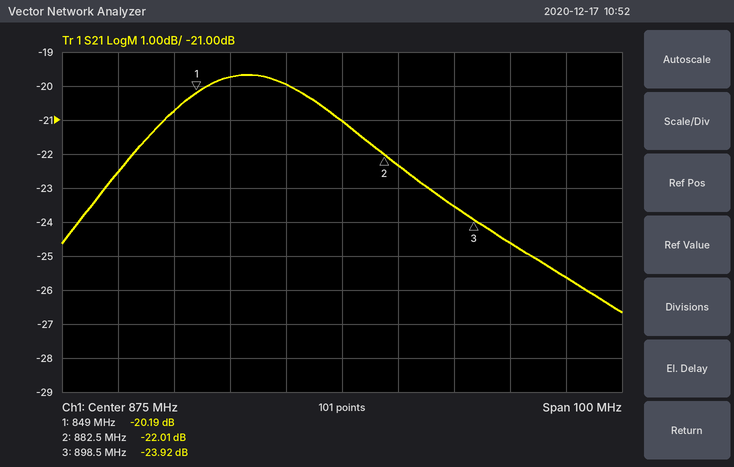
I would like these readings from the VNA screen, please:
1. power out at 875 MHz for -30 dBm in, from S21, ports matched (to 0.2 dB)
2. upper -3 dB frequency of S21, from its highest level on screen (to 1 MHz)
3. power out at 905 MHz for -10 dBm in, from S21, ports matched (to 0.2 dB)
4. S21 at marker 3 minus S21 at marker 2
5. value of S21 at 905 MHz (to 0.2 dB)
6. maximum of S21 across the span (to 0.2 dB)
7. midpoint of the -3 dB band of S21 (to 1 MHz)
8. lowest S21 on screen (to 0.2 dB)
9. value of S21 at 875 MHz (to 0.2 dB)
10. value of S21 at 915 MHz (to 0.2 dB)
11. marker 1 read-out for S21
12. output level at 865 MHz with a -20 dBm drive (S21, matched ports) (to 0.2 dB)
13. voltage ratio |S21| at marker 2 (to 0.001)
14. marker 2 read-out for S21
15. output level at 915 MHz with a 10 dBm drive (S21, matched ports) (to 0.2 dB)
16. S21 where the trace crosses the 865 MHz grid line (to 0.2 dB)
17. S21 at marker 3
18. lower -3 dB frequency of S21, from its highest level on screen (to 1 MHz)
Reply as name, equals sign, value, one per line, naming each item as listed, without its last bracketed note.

power out at 875 MHz for -30 dBm in, from S21, ports matched = -51.0 dBm
upper -3 dB frequency of S21, from its highest level on screen = 888 MHz
power out at 905 MHz for -10 dBm in, from S21, ports matched = -34.6 dBm
S21 at marker 3 minus S21 at marker 2 = -1.91 dB
value of S21 at 905 MHz = -24.6 dB
maximum of S21 across the span = -19.6 dB
midpoint of the -3 dB band of S21 = 861 MHz
lowest S21 on screen = -26.6 dB
value of S21 at 875 MHz = -21.0 dB
value of S21 at 915 MHz = -25.6 dB
marker 1 read-out for S21 = -20.19 dB
output level at 865 MHz with a -20 dBm drive (S21, matched ports) = -40.0 dBm
voltage ratio |S21| at marker 2 = 0.079
marker 2 read-out for S21 = -22.01 dB
output level at 915 MHz with a 10 dBm drive (S21, matched ports) = -15.6 dBm
S21 where the trace crosses the 865 MHz grid line = -20.0 dB
S21 at marker 3 = -23.92 dB
lower -3 dB frequency of S21, from its highest level on screen = 834 MHz
